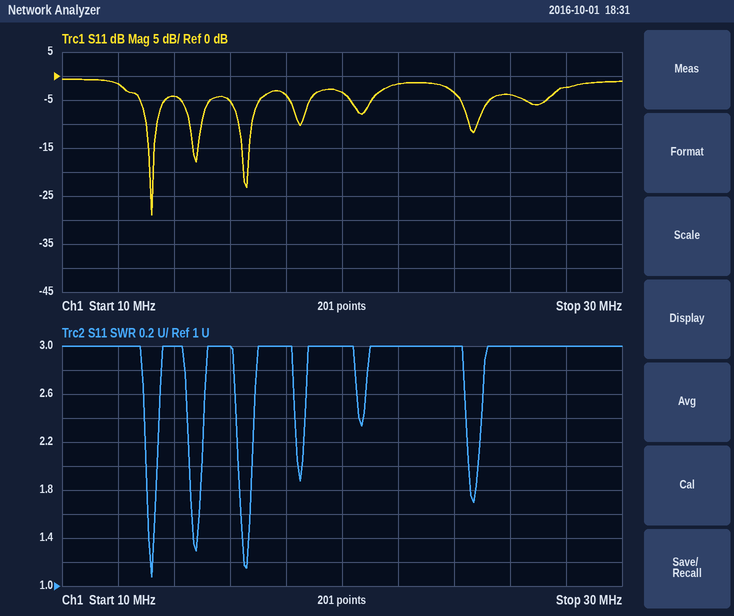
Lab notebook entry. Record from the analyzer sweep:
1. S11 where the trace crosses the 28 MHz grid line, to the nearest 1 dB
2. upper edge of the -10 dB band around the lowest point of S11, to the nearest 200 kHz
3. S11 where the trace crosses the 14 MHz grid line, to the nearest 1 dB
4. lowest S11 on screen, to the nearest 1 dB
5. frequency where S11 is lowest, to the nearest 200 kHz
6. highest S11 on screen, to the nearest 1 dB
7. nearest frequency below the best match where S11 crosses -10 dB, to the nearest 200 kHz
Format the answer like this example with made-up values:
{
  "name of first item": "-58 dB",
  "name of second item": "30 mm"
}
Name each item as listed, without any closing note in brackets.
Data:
{
  "S11 where the trace crosses the 28 MHz grid line, to the nearest 1 dB": "-2 dB",
  "upper edge of the -10 dB band around the lowest point of S11, to the nearest 200 kHz": "13.4 MHz",
  "S11 where the trace crosses the 14 MHz grid line, to the nearest 1 dB": "-4 dB",
  "lowest S11 on screen, to the nearest 1 dB": "-29 dB",
  "frequency where S11 is lowest, to the nearest 200 kHz": "13.2 MHz",
  "highest S11 on screen, to the nearest 1 dB": "-1 dB",
  "nearest frequency below the best match where S11 crosses -10 dB, to the nearest 200 kHz": "13.0 MHz"
}
